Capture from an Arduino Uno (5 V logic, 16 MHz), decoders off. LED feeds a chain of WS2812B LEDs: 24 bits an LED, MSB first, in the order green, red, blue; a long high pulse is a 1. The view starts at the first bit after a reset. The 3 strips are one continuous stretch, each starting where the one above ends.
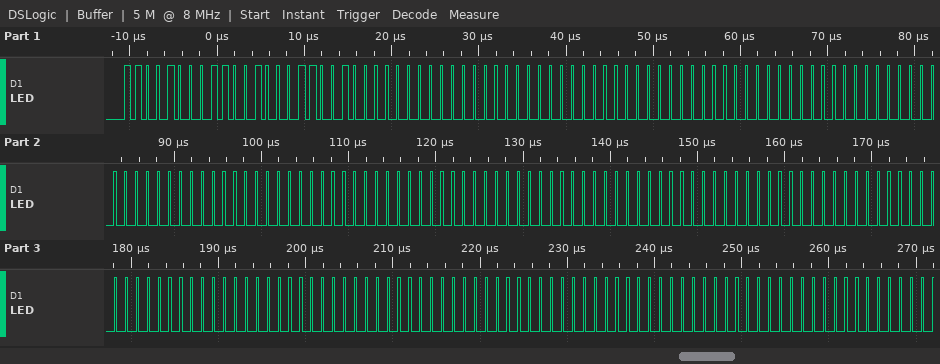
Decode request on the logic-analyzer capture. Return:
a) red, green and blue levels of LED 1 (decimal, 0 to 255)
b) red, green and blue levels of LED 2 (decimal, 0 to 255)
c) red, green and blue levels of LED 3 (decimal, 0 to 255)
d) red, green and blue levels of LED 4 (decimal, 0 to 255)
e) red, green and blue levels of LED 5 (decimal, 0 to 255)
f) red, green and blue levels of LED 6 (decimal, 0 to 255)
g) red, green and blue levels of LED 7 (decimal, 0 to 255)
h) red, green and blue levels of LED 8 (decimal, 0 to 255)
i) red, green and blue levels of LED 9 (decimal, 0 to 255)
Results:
200, 200, 200
0, 0, 0
0, 0, 0
0, 0, 0
0, 0, 0
0, 0, 0
0, 0, 0
0, 0, 0
0, 0, 0
